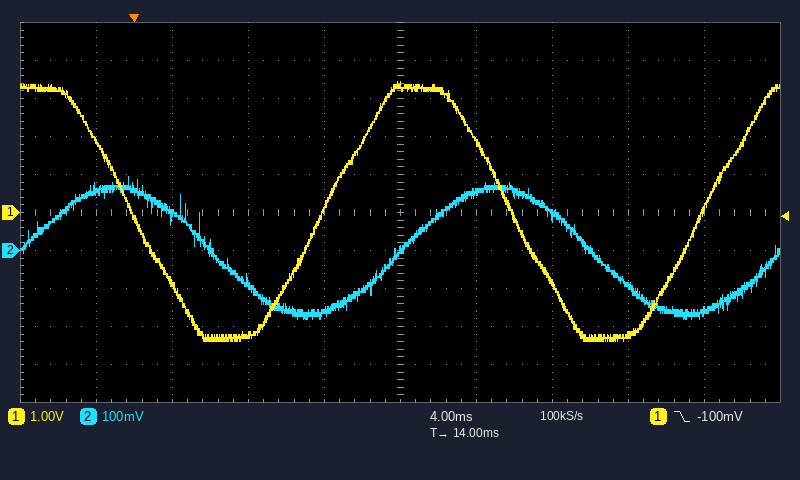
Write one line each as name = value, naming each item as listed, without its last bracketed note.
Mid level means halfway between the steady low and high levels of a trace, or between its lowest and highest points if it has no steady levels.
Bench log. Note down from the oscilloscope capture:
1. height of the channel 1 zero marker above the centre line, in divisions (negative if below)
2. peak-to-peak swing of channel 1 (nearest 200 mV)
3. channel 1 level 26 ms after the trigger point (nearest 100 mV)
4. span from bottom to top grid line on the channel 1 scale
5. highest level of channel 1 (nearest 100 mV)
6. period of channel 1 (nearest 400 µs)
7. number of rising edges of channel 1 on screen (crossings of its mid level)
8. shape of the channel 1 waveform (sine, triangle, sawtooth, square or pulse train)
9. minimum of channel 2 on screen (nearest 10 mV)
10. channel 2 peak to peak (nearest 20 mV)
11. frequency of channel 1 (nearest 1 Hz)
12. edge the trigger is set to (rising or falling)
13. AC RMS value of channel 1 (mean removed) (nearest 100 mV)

height of the channel 1 zero marker above the centre line, in divisions = 0.0 div
peak-to-peak swing of channel 1 = 6.8 V
channel 1 level 26 ms after the trigger point = -3.2 V
span from bottom to top grid line on the channel 1 scale = 10 V
highest level of channel 1 = 3.4 V
period of channel 1 = 20.0 ms
number of rising edges of channel 1 on screen = 2
shape of the channel 1 waveform = sine
minimum of channel 2 on screen = -180 mV
channel 2 peak to peak = 380 mV
frequency of channel 1 = 50 Hz
edge the trigger is set to = falling
AC RMS value of channel 1 (mean removed) = 2.4 V
